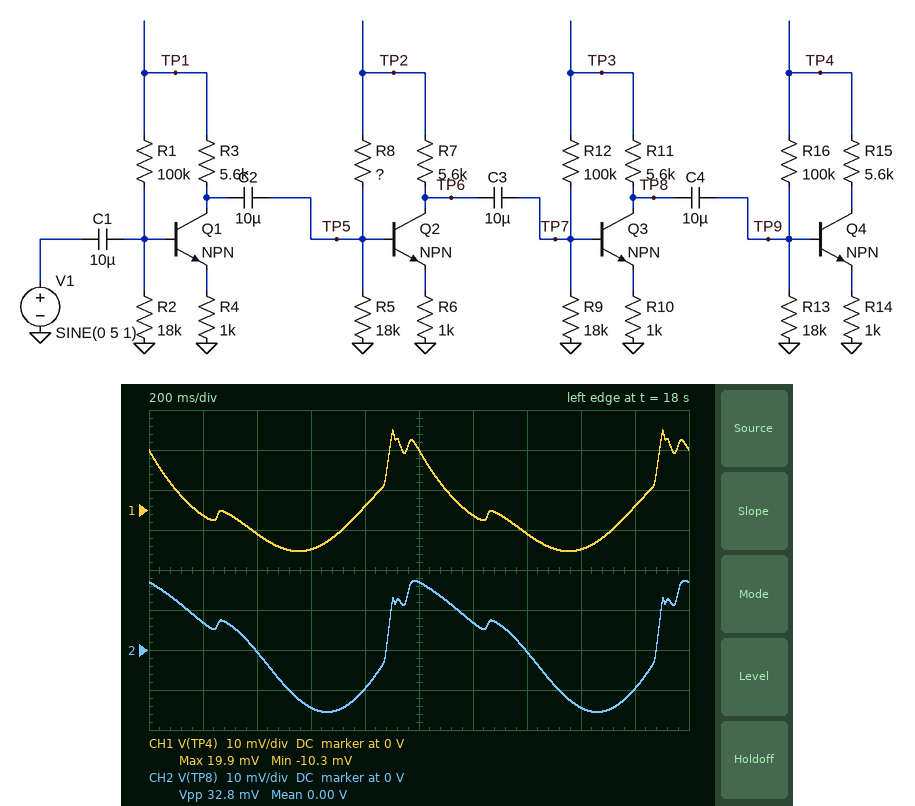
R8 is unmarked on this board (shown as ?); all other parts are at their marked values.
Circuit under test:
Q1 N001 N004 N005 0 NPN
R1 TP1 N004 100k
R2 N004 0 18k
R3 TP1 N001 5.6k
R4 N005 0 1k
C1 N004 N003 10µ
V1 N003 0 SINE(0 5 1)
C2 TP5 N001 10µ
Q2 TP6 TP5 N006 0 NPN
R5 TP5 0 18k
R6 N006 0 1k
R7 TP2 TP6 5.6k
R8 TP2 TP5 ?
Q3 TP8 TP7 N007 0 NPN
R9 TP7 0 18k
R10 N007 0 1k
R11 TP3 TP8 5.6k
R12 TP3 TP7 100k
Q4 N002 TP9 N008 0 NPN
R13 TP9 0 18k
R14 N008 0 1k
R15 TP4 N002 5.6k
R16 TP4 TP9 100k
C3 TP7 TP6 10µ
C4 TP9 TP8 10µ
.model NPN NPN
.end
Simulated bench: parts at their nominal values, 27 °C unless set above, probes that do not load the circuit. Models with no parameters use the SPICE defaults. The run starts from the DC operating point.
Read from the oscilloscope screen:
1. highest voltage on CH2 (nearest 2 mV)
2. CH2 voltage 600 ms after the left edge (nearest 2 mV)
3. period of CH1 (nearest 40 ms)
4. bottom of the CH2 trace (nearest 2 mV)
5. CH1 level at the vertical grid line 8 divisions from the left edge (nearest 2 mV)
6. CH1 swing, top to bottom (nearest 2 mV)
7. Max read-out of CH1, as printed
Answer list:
18 mV
-14 mV
1.00 s
-16 mV
-10 mV
30 mV
19.9 mV
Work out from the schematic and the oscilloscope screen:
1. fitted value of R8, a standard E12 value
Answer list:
56 kΩ
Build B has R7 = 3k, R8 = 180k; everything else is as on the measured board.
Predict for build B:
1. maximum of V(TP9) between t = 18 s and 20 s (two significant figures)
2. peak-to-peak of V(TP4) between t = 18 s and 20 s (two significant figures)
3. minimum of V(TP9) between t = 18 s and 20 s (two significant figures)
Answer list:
12 mV
17 mV
-4.7 mV
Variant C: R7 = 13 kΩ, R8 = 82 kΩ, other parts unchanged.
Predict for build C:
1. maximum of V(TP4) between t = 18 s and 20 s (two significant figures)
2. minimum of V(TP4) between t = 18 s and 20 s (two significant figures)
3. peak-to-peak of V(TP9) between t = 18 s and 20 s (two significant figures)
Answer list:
16 mV
-7.8 mV
23 mV
